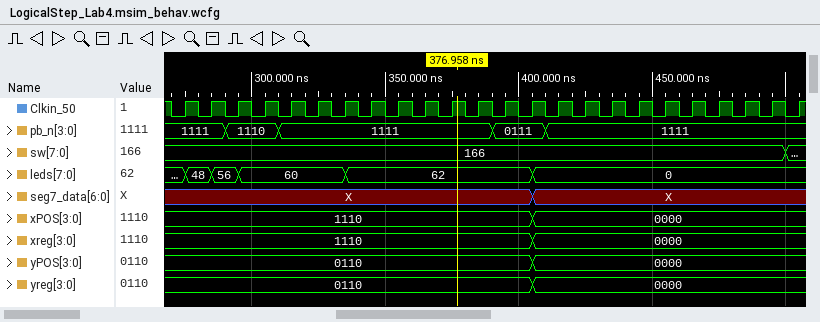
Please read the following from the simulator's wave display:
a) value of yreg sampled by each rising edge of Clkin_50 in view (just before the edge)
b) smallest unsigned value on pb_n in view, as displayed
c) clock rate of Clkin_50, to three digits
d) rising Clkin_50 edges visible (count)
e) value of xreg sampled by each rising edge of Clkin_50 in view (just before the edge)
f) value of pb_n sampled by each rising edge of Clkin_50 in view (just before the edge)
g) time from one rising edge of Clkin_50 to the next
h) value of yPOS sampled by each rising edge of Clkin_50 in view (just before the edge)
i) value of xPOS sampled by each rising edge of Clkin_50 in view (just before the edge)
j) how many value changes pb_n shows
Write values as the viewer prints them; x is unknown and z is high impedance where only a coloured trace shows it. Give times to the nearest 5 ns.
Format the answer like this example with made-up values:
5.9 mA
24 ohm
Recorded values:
0110, 0110, 0110, 0110, 0110, 0110, 0110, 0110, 0110, 0110, 0110, 0110, 0110, 0110, 0000, 0000, 0000, 0000, 0000, 0000, 0000, 0000, 0000, 0000
0111
100 MHz
24
1110, 1110, 1110, 1110, 1110, 1110, 1110, 1110, 1110, 1110, 1110, 1110, 1110, 1110, 0000, 0000, 0000, 0000, 0000, 0000, 0000, 0000, 0000, 0000
1111, 1111, 1110, 1110, 1111, 1111, 1111, 1111, 1111, 1111, 1111, 1111, 0111, 0111, 1111, 1111, 1111, 1111, 1111, 1111, 1111, 1111, 1111, 1111
10 ns
0110, 0110, 0110, 0110, 0110, 0110, 0110, 0110, 0110, 0110, 0110, 0110, 0110, 0110, 0000, 0000, 0000, 0000, 0000, 0000, 0000, 0000, 0000, 0000
1110, 1110, 1110, 1110, 1110, 1110, 1110, 1110, 1110, 1110, 1110, 1110, 1110, 1110, 0000, 0000, 0000, 0000, 0000, 0000, 0000, 0000, 0000, 0000
4
